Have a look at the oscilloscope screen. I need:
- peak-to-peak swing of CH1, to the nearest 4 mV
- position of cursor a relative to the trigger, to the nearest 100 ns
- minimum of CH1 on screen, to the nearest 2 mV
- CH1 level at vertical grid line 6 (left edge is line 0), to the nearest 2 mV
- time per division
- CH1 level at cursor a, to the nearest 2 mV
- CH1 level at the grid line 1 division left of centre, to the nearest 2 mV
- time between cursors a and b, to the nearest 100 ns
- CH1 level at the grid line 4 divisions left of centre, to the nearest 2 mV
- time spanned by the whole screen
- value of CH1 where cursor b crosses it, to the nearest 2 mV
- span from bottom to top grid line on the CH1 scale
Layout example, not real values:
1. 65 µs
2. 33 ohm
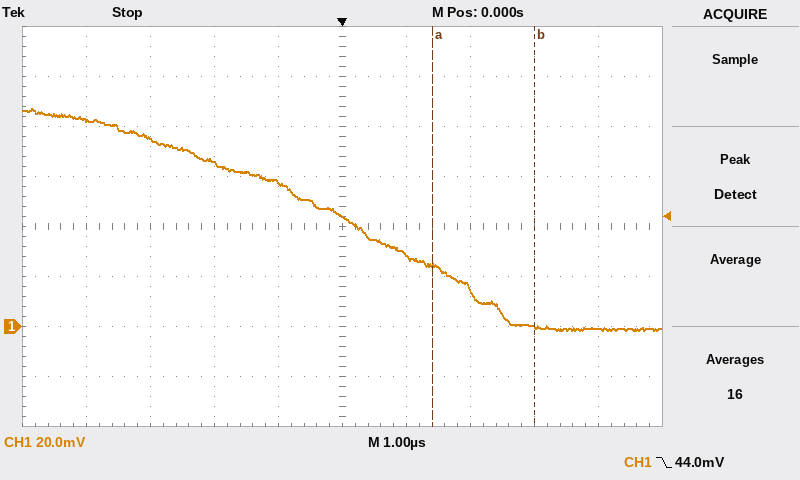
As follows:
1. 88 mV
2. +1.4 µs
3. -2 mV
4. 28 mV
5. 1 µs
6. 24 mV
7. 58 mV
8. 1.6 µs
9. 82 mV
10. 10 µs
11. 0 mV
12. 160 mV
